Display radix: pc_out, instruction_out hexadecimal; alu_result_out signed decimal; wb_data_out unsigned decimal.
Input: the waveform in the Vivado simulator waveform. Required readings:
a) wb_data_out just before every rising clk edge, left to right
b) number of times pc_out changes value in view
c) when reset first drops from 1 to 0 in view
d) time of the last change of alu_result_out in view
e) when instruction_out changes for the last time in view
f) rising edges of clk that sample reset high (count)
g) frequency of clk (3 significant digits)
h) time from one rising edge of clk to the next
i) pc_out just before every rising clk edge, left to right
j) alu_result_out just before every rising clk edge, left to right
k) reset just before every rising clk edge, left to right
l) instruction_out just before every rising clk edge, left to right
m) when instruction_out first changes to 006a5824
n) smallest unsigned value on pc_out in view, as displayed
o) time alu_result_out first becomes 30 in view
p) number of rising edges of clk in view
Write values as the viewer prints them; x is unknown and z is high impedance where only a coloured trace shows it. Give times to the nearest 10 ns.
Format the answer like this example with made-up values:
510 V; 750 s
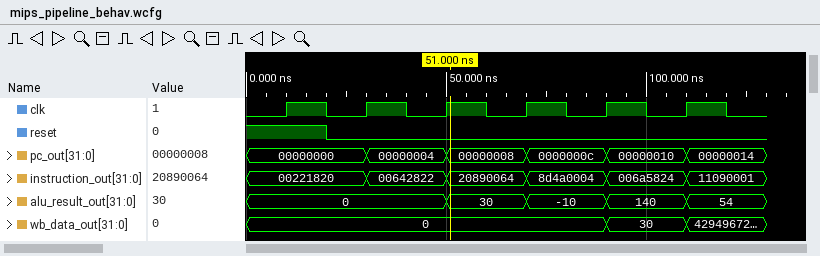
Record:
0, 0, 0, 0, 0, 30; 5; 20 ns; 110 ns; 110 ns; 1; 50.0 MHz; 20 ns; 00000000, 00000000, 00000004, 00000008, 0000000c, 00000010; 0, 0, 0, 30, -10, 140; 1 0 0 0 0 0; 00221820, 00221820, 00642822, 20890064, 8d4a0004, 006a5824; 90 ns; 00000000; 50 ns; 6
